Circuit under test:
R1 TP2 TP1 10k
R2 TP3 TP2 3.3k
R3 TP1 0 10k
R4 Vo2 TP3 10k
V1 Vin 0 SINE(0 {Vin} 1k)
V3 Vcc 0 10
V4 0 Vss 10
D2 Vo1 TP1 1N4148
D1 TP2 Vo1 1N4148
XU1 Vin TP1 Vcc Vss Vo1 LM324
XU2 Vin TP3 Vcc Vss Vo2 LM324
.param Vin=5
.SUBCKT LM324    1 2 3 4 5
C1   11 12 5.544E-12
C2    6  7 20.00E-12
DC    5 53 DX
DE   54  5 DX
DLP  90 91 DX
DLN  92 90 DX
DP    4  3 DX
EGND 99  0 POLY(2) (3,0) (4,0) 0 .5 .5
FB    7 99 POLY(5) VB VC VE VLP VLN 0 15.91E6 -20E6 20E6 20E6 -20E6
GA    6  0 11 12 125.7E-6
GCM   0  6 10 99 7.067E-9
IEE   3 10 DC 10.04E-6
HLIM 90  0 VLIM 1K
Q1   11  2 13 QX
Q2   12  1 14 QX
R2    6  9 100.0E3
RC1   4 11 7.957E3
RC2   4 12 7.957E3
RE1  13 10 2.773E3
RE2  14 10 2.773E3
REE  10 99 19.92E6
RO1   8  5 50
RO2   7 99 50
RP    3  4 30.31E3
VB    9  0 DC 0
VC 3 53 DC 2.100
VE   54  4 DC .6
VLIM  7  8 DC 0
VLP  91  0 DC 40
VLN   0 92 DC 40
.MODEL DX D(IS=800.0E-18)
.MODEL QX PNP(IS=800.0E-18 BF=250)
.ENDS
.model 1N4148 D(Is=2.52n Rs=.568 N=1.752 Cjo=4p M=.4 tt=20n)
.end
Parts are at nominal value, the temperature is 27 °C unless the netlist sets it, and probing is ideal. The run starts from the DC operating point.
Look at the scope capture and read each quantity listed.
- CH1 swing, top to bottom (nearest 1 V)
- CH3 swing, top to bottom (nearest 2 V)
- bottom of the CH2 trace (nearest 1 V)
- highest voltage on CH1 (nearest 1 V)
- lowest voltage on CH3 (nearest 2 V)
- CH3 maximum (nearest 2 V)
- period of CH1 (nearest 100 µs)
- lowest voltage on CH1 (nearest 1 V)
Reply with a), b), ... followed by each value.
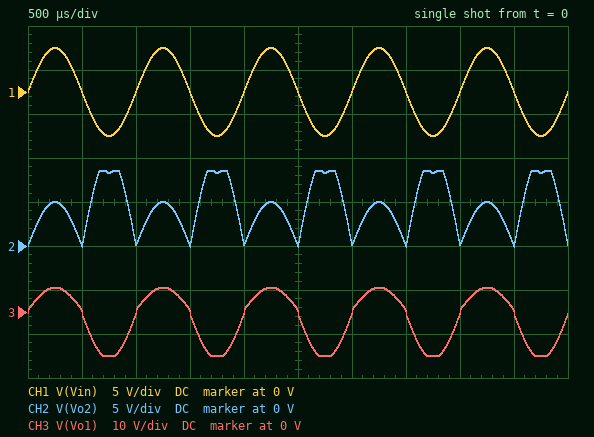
a) 10 V
b) 16 V
c) 0 V
d) 5 V
e) -10 V
f) 6 V
g) 1.0 ms
h) -5 V
